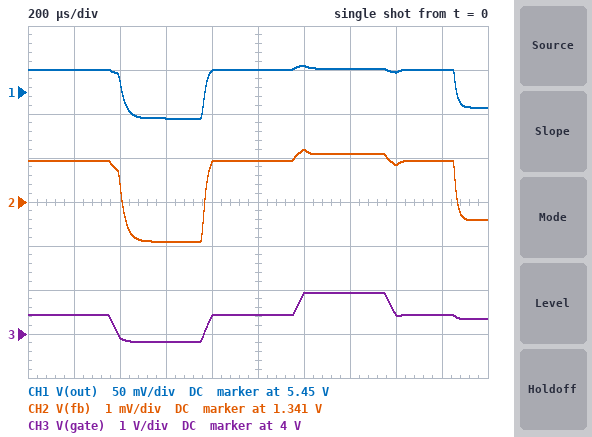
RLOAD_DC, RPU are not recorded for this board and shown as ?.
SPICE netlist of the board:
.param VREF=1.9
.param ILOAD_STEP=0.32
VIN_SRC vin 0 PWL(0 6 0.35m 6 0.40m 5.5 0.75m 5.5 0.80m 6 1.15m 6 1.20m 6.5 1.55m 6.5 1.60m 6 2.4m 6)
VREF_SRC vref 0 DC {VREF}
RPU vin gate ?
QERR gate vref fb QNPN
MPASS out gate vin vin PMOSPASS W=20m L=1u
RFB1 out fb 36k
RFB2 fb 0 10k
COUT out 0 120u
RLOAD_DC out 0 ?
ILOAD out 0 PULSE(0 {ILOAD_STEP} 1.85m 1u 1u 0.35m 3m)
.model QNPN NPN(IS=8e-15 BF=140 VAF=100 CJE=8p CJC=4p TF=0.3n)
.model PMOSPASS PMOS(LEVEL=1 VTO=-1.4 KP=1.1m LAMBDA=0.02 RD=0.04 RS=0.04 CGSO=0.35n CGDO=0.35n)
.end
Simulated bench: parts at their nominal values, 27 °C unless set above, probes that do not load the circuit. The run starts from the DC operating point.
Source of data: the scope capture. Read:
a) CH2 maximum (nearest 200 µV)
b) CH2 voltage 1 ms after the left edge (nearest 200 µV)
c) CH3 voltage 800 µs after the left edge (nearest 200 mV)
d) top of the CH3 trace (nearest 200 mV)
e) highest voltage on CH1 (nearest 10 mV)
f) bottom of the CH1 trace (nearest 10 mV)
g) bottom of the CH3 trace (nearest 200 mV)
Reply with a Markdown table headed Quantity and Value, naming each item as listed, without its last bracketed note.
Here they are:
| Quantity | Value |
|---|---|
| CH2 maximum | 1.3422 V |
| CH2 voltage 1 ms after the left edge | 1.3420 V |
| CH3 voltage 800 µs after the left edge | 4.4 V |
| top of the CH3 trace | 5.0 V |
| highest voltage on CH1 | 5.48 V |
| bottom of the CH1 trace | 5.42 V |
| bottom of the CH3 trace | 3.8 V |
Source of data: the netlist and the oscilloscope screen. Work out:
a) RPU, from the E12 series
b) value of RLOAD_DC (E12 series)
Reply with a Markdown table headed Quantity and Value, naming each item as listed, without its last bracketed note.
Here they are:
| Quantity | Value |
|---|---|
| RPU, from the E12 series | 82 kΩ |
| value of RLOAD_DC | 18 Ω |
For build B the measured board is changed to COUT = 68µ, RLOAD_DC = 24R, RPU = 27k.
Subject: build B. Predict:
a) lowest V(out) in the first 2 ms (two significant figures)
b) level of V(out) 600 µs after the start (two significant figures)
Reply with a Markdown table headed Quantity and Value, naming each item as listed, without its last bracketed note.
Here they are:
| Quantity | Value |
|---|---|
| lowest V(out) in the first 2 ms | 3.9 V |
| level of V(out) 600 µs after the start | 4.0 V |
